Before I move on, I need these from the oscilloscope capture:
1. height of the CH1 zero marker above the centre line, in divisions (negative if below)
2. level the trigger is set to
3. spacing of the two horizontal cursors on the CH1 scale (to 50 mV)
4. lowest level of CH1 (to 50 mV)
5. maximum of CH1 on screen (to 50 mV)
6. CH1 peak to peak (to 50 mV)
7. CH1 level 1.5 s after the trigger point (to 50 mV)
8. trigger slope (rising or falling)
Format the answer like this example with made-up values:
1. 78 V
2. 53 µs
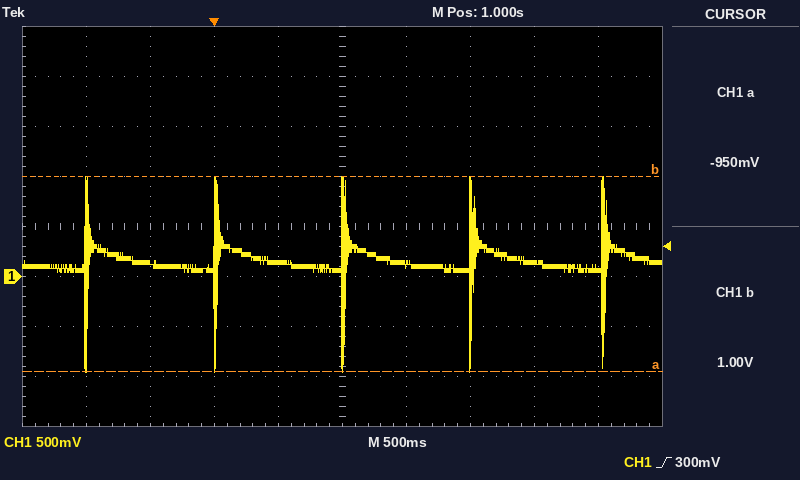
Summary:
1. -1.0 div
2. 300 mV
3. 1.95 V
4. -950 mV
5. 1.00 V
6. 1.95 V
7. 100 mV
8. rising
